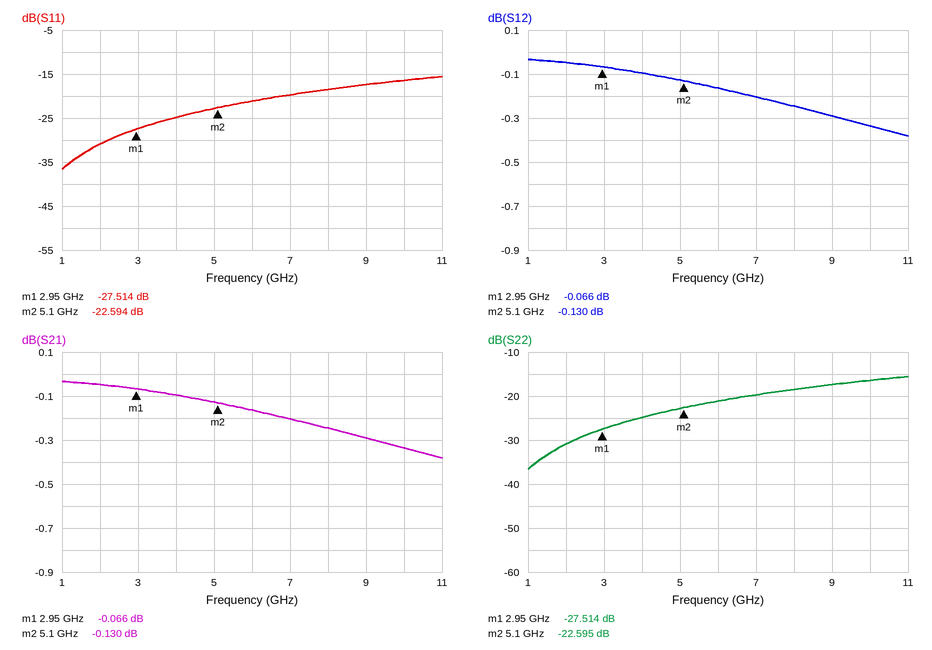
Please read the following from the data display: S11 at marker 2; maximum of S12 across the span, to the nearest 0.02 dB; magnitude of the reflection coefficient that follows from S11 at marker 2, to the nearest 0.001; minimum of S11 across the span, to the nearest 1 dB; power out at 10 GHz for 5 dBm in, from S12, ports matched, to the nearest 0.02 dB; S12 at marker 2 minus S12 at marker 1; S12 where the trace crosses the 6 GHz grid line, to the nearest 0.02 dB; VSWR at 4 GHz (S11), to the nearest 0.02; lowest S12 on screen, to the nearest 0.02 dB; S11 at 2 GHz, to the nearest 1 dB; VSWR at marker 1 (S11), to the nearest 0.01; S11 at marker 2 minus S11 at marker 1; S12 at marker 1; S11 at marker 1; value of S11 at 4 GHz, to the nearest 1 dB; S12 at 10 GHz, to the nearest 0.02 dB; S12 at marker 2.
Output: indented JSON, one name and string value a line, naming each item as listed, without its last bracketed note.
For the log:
{
  "S11 at marker 2": "-22.594 dB",
  "maximum of S12 across the span, to the nearest 0.02 dB": "-0.04 dB",
  "magnitude of the reflection coefficient that follows from S11 at marker 2, to the nearest 0.001": "0.074",
  "minimum of S11 across the span, to the nearest 1 dB": "-37 dB",
  "power out at 10 GHz for 5 dBm in, from S12, ports matched, to the nearest 0.02 dB": "4.66 dBm",
  "S12 at marker 2 minus S12 at marker 1": "-0.064 dB",
  "S12 where the trace crosses the 6 GHz grid line, to the nearest 0.02 dB": "-0.16 dB",
  "VSWR at 4 GHz (S11), to the nearest 0.02": "1.12",
  "lowest S12 on screen, to the nearest 0.02 dB": "-0.38 dB",
  "S11 at 2 GHz, to the nearest 1 dB": "-31 dB",
  "VSWR at marker 1 (S11), to the nearest 0.01": "1.09",
  "S11 at marker 2 minus S11 at marker 1": "4.920 dB",
  "S12 at marker 1": "-0.066 dB",
  "S11 at marker 1": "-27.514 dB",
  "value of S11 at 4 GHz, to the nearest 1 dB": "-25 dB",
  "S12 at 10 GHz, to the nearest 0.02 dB": "-0.34 dB",
  "S12 at marker 2": "-0.130 dB"
}
